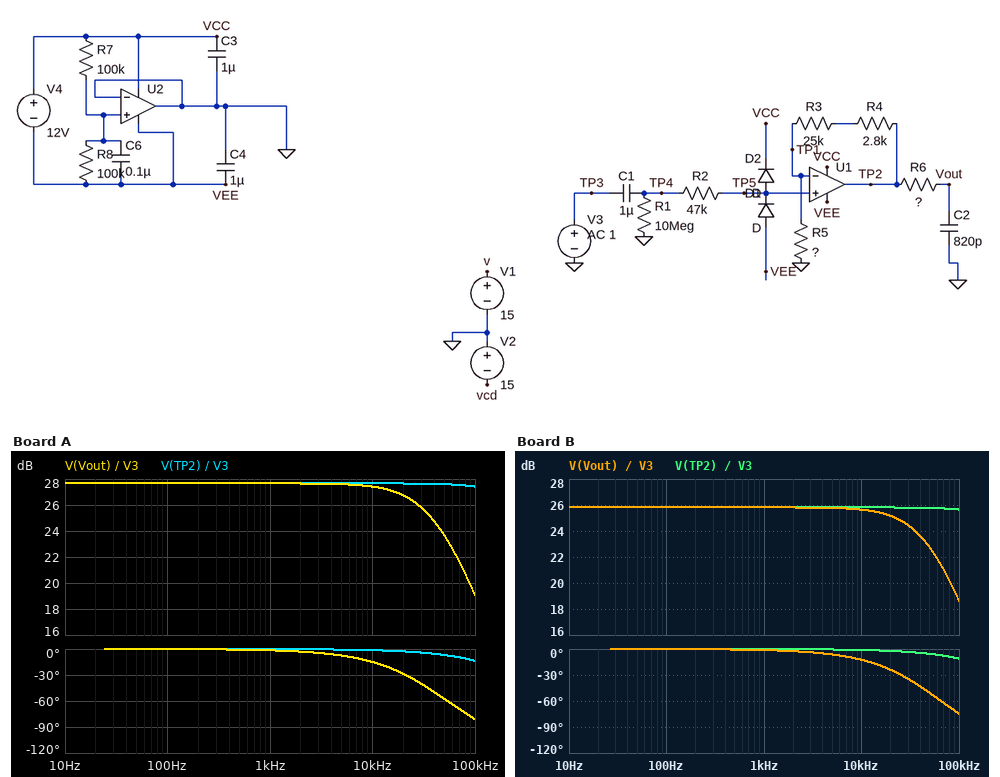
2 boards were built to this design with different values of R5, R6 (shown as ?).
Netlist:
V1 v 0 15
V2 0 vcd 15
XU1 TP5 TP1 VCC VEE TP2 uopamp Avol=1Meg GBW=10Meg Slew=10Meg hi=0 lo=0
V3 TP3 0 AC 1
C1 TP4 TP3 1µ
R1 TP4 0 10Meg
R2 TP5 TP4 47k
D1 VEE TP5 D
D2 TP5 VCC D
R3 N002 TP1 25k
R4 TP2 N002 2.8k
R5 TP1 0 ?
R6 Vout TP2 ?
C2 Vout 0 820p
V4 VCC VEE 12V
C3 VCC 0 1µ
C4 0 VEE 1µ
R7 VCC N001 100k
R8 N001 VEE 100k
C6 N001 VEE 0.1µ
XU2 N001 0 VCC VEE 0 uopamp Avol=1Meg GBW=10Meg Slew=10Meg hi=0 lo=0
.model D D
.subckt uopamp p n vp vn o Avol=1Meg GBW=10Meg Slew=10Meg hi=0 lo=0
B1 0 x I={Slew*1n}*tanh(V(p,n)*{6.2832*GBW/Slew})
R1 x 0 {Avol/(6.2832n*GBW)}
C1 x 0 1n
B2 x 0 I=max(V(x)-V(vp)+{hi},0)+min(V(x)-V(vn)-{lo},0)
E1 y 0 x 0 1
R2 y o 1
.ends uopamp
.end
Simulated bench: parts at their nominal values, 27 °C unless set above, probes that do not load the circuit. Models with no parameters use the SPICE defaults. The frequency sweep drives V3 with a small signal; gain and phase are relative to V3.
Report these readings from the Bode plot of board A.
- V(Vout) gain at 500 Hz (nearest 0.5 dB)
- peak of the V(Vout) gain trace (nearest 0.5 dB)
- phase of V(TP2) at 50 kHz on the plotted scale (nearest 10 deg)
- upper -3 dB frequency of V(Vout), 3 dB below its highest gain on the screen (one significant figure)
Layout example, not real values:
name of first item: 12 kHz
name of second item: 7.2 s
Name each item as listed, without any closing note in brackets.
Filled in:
V(Vout) gain at 500 Hz: 27.5 dB
peak of the V(Vout) gain trace: 27.5 dB
phase of V(TP2) at 50 kHz on the plotted scale: -10 deg
upper -3 dB frequency of V(Vout), 3 dB below its highest gain on the screen: 40 kHz
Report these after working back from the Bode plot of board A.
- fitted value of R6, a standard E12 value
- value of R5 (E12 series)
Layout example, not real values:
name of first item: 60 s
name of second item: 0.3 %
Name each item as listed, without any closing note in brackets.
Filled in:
fitted value of R6, a standard E12 value: 4.7 kΩ
value of R5: 1.2 kΩ
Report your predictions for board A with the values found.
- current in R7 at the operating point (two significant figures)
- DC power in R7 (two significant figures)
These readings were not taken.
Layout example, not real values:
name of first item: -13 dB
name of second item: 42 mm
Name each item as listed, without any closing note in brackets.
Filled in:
current in R7 at the operating point: 60 µA
DC power in R7: 360 µW
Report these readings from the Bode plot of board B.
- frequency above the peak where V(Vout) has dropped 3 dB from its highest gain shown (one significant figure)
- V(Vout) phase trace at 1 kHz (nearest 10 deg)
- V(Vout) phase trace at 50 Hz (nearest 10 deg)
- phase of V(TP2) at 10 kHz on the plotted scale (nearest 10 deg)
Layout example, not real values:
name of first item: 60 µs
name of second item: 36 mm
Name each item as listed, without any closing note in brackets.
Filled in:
frequency above the peak where V(Vout) has dropped 3 dB from its highest gain shown: 50 kHz
V(Vout) phase trace at 1 kHz: 0 deg
V(Vout) phase trace at 50 Hz: 0 deg
phase of V(TP2) at 10 kHz on the plotted scale: 0 deg
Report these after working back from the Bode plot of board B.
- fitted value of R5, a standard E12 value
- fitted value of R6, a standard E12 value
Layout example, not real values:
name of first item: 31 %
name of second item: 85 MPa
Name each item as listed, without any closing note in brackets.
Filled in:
fitted value of R5, a standard E12 value: 1.5 kΩ
fitted value of R6, a standard E12 value: 3.9 kΩ
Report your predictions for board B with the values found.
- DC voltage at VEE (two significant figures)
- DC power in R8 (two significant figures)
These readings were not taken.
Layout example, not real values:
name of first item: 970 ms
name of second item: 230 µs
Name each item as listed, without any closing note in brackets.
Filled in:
DC voltage at VEE: -6.0 V
DC power in R8: 360 µW
